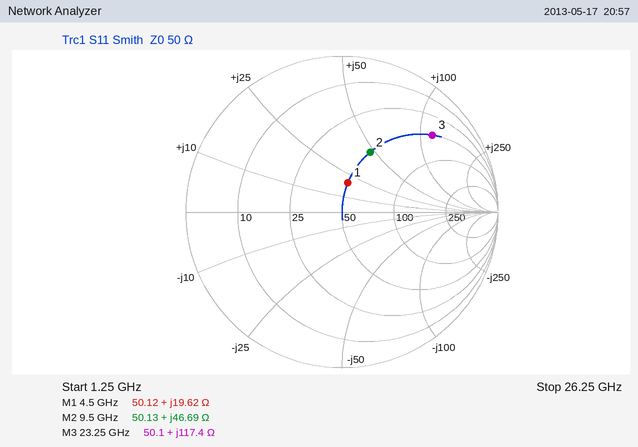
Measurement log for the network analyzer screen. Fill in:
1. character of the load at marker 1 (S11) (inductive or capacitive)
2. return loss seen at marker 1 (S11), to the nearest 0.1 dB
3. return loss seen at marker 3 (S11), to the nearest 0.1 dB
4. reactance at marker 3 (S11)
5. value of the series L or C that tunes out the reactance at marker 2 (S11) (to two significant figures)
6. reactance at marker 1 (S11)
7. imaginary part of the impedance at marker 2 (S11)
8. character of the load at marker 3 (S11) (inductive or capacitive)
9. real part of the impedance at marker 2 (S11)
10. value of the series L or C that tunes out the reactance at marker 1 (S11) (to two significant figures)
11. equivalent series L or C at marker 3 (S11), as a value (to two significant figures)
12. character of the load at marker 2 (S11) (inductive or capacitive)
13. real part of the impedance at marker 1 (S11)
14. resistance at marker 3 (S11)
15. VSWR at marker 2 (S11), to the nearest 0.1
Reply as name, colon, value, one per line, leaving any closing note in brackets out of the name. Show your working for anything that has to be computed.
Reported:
character of the load at marker 1 (S11): inductive
return loss seen at marker 1 (S11), to the nearest 0.1 dB: 14.3 dB
return loss seen at marker 3 (S11), to the nearest 0.1 dB: 2.4 dB
reactance at marker 3: +117.4 Ω
value of the series L or C that tunes out the reactance at marker 2 (S11): C = 1/(2π × 9.5 GHz × 46.69 Ω) ≈ 359 fF, so 360 fF to two significant figures
reactance at marker 1: +19.62 Ω
imaginary part of the impedance at marker 2: +46.69 Ω
character of the load at marker 3 (S11): inductive
real part of the impedance at marker 2: 50.13 Ω
value of the series L or C that tunes out the reactance at marker 1 (S11): C = 1/(2π × 4.5 GHz × 19.62 Ω) ≈ 1.8 pF
equivalent series L or C at marker 3 (S11), as a value: L = 117.4 Ω/(2π × 23.25 GHz) ≈ 804 pH, so 800 pH to two significant figures
character of the load at marker 2 (S11): inductive
real part of the impedance at marker 1: 50.12 Ω
resistance at marker 3: 50.1 Ω
VSWR at marker 2 (S11), to the nearest 0.1: 2.5
